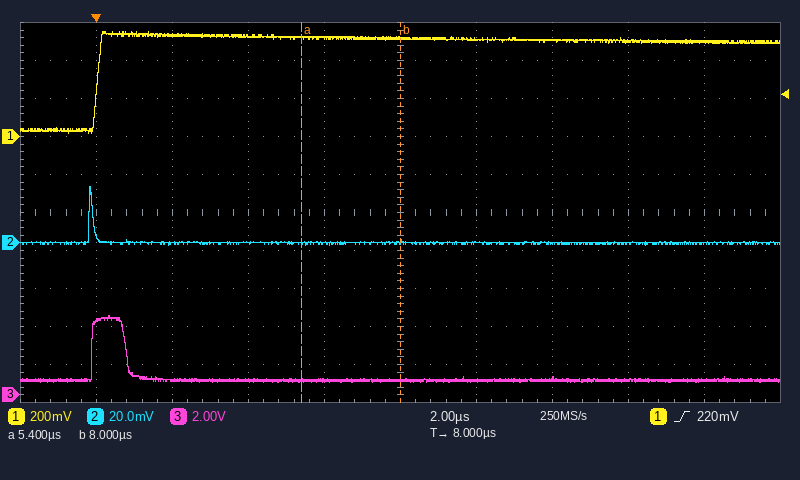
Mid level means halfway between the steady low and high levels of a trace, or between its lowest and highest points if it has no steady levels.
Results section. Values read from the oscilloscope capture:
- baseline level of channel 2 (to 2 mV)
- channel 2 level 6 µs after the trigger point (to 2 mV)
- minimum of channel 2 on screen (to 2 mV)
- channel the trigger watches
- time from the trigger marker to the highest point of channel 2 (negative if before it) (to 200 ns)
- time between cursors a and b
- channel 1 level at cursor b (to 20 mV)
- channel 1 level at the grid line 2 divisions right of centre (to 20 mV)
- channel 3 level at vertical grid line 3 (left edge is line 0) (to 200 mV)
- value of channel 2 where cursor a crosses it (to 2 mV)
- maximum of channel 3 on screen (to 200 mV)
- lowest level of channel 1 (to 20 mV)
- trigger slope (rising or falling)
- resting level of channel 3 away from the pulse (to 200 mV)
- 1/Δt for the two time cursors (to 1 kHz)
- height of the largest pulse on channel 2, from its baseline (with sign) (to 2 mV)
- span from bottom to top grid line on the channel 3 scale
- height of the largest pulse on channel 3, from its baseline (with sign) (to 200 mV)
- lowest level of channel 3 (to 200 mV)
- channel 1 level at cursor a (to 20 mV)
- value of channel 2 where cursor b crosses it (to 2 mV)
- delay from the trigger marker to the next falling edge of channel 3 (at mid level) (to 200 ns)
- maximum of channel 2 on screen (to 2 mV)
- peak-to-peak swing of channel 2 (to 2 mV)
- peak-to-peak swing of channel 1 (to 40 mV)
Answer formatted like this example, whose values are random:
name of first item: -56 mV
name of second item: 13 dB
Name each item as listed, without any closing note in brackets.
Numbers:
baseline level of channel 2: 0 mV
channel 2 level 6 µs after the trigger point: 0 mV
minimum of channel 2 on screen: -2 mV
channel the trigger watches: channel 1
time from the trigger marker to the highest point of channel 2 (negative if before it): -200 ns
time between cursors a and b: 2.6 µs
channel 1 level at cursor b: 520 mV
channel 1 level at the grid line 2 divisions right of centre: 500 mV
channel 3 level at vertical grid line 3 (left edge is line 0): 800 mV
value of channel 2 where cursor a crosses it: 0 mV
maximum of channel 3 on screen: 4.2 V
lowest level of channel 1: 20 mV
trigger slope: rising
resting level of channel 3 away from the pulse: 800 mV
1/Δt for the two time cursors: 385 kHz
height of the largest pulse on channel 2, from its baseline (with sign): +30 mV
span from bottom to top grid line on the channel 3 scale: 20 V
height of the largest pulse on channel 3, from its baseline (with sign): +3.4 V
lowest level of channel 3: 600 mV
channel 1 level at cursor a: 520 mV
value of channel 2 where cursor b crosses it: 0 mV
delay from the trigger marker to the next falling edge of channel 3 (at mid level): 800 ns
maximum of channel 2 on screen: 30 mV
peak-to-peak swing of channel 2: 32 mV
peak-to-peak swing of channel 1: 520 mV
